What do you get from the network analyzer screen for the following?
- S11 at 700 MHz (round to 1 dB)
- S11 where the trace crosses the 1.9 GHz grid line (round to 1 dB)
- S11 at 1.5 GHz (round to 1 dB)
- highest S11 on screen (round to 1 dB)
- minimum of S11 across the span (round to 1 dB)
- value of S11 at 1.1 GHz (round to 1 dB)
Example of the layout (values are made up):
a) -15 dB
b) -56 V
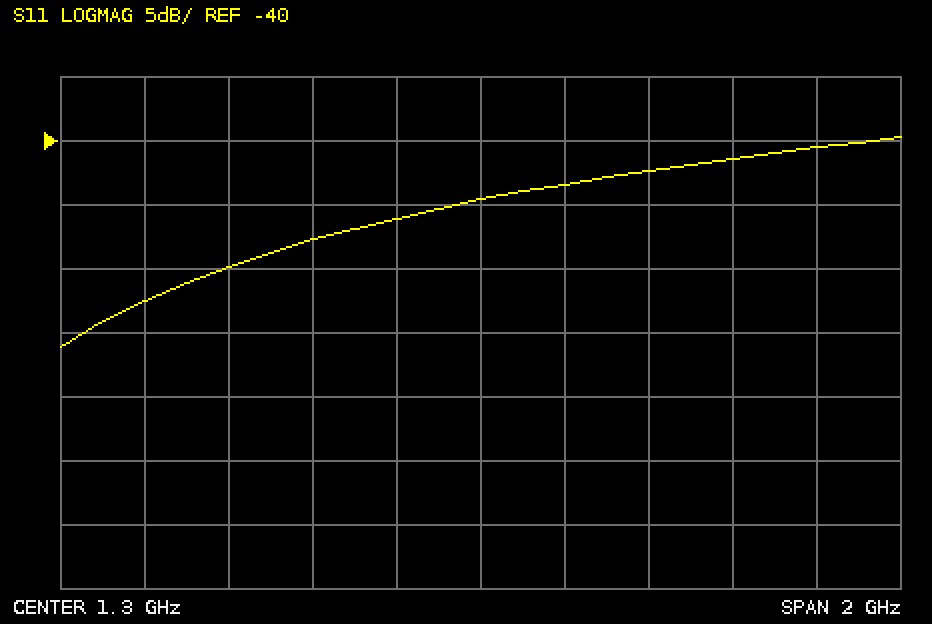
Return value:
a) -50 dB
b) -41 dB
c) -43 dB
d) -40 dB
e) -56 dB
f) -46 dB
